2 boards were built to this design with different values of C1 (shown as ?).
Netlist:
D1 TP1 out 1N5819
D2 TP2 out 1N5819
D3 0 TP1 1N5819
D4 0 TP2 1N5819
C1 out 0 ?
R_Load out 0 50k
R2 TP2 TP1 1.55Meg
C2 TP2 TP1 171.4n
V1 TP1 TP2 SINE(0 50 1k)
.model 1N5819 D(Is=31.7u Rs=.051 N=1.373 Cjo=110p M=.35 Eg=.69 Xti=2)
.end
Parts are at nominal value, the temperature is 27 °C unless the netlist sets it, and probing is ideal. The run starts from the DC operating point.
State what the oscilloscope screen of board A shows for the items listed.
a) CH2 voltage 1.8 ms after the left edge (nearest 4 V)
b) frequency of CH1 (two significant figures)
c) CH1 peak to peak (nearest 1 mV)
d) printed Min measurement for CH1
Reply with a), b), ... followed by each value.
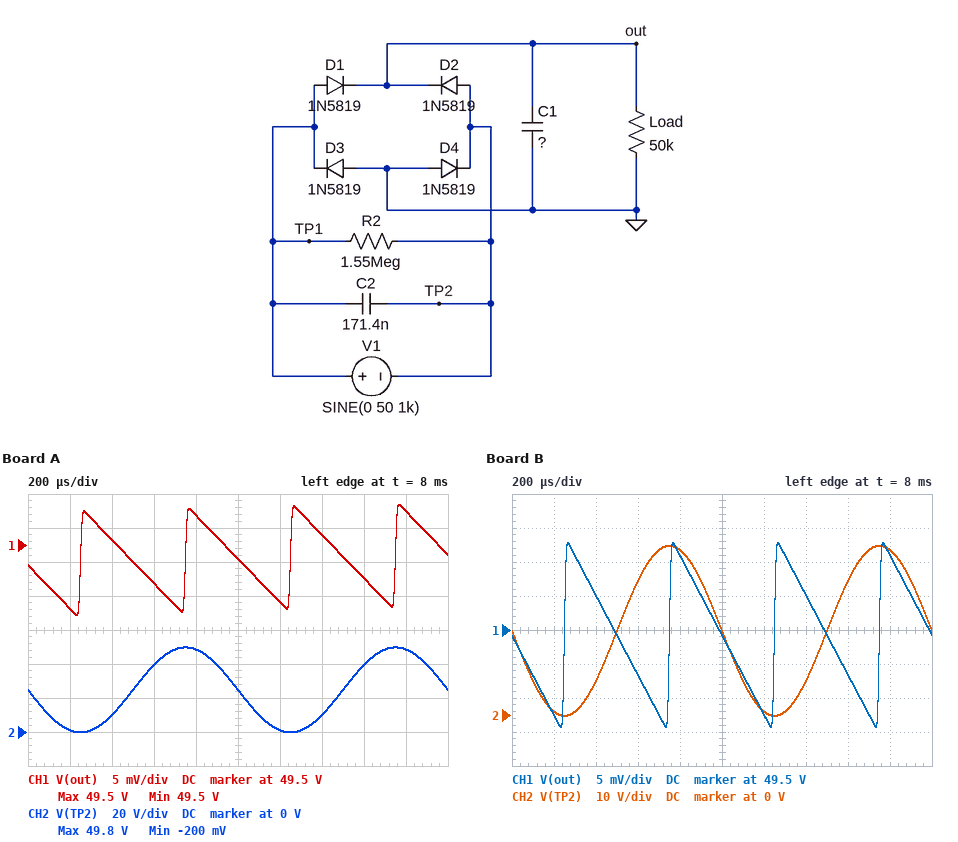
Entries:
a) 48 V
b) 2.0 kHz
c) 16 mV
d) 49.5 V
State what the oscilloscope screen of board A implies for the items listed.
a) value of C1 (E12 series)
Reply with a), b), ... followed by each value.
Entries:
a) 33 µF
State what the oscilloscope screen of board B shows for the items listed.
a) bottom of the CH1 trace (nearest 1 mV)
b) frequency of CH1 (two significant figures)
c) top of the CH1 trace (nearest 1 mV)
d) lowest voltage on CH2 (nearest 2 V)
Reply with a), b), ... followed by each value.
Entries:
a) 49.486 V
b) 2.0 kHz
c) 49.513 V
d) 0 V
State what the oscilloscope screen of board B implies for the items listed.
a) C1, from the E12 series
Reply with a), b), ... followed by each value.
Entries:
a) 18 µF
